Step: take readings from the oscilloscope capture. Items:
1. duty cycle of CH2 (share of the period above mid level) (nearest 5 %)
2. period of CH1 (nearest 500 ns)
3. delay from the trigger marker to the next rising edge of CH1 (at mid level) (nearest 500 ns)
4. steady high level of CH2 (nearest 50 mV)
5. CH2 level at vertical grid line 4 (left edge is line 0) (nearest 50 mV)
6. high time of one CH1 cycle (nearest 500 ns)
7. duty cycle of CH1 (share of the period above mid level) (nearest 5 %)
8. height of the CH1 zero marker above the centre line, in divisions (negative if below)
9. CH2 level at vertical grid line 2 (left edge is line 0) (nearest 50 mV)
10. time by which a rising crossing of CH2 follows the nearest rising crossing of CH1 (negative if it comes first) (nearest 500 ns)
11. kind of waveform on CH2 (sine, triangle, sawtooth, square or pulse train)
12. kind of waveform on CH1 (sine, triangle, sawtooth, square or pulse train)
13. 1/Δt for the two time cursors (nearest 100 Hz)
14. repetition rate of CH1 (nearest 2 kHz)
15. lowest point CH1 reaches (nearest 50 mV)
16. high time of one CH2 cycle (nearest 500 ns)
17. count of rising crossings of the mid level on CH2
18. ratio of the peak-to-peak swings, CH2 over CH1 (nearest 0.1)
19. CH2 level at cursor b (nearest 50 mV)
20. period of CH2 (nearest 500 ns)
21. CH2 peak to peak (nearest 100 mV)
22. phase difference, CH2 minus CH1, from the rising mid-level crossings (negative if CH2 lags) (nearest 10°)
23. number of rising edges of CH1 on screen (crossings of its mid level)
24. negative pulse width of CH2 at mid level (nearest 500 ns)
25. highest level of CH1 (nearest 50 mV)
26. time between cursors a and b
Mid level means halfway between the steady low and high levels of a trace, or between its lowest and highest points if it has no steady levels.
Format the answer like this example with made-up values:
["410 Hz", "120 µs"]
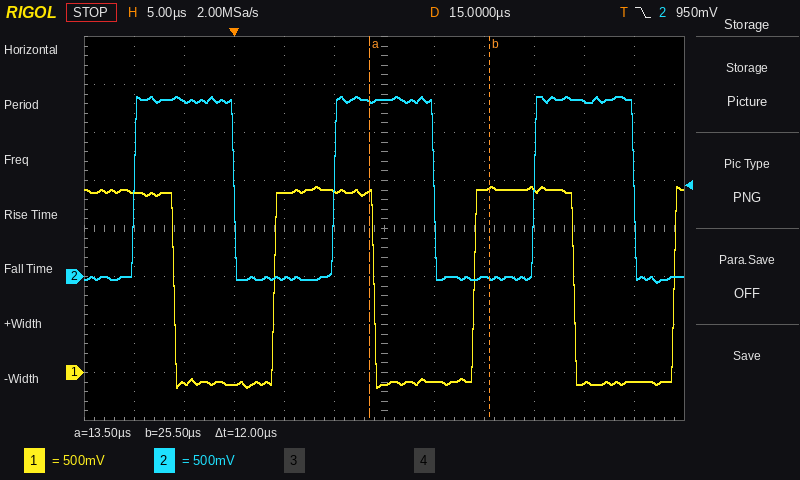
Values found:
["50 %", "20.0 µs", "4.0 µs", "1.85 V", "0 mV", "10.0 µs", "50 %", "-3.0 div", "1.85 V", "+6.0 µs", "square", "square", "83.3 kHz", "50 kHz", "-150 mV", "10.0 µs", "3", "0.9", "0 mV", "20.0 µs", "1.90 V", "-110°", "3", "10.0 µs", "1.95 V", "12 µs"]
